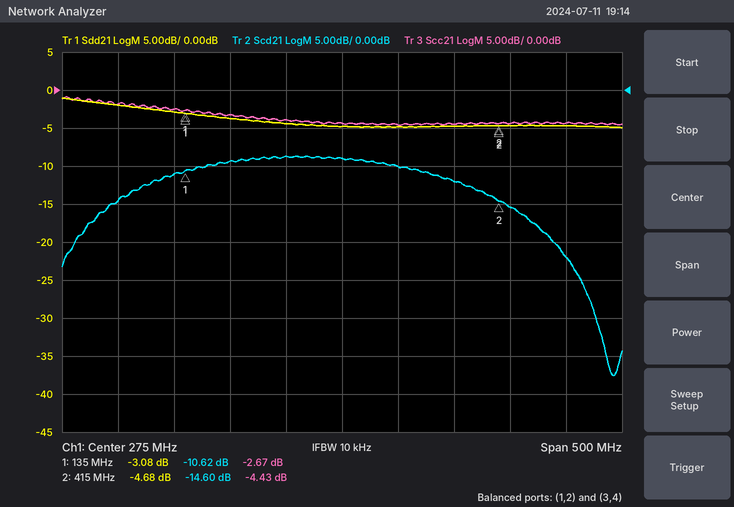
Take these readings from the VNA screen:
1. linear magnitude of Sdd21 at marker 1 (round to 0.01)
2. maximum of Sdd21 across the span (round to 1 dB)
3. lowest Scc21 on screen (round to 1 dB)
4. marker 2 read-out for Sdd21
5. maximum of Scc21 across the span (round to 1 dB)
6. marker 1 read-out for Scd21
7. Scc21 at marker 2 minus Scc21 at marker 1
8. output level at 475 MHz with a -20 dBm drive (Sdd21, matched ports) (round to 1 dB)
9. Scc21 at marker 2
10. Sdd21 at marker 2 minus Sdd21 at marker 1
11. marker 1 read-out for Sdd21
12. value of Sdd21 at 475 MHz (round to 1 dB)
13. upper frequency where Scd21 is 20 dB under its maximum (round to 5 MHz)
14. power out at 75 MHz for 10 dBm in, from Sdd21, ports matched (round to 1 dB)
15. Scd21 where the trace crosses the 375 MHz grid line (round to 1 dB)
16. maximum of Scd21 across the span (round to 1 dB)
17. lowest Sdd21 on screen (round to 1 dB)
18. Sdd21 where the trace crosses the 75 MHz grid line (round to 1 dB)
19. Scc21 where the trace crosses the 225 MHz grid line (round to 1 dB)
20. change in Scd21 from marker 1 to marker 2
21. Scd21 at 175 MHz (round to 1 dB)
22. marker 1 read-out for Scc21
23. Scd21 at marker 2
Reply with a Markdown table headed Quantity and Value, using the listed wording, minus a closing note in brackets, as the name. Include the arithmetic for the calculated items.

| Quantity | Value |
|---|---|
| linear magnitude of Sdd21 at marker 1 | 10^(-3.08/20) ≈ 0.70 |
| maximum of Sdd21 across the span | -1 dB |
| lowest Scc21 on screen | -5 dB |
| marker 2 read-out for Sdd21 | -4.68 dB |
| maximum of Scc21 across the span | -1 dB |
| marker 1 read-out for Scd21 | -10.62 dB |
| Scc21 at marker 2 minus Scc21 at marker 1 | -4.43 − (-2.67) = -1.76 dB |
| output level at 475 MHz with a -20 dBm drive (Sdd21, matched ports) | -20 dBm + (-5 dB) = -25 dBm |
| Scc21 at marker 2 | -4.43 dB |
| Sdd21 at marker 2 minus Sdd21 at marker 1 | -4.68 − (-3.08) = -1.60 dB |
| marker 1 read-out for Sdd21 | -3.08 dB |
| value of Sdd21 at 475 MHz | -5 dB |
| upper frequency where Scd21 is 20 dB under its maximum | 500 MHz |
| power out at 75 MHz for 10 dBm in, from Sdd21, ports matched | 10 dBm + (-2 dB) = 8 dBm |
| Scd21 where the trace crosses the 375 MHz grid line | -12 dB |
| maximum of Scd21 across the span | -9 dB |
| lowest Sdd21 on screen | -5 dB |
| Sdd21 where the trace crosses the 75 MHz grid line | -2 dB |
| Scc21 where the trace crosses the 225 MHz grid line | -4 dB |
| change in Scd21 from marker 1 to marker 2 | -14.6 − (-10.62) = -3.98 dB |
| Scd21 at 175 MHz | -9 dB |
| marker 1 read-out for Scc21 | -2.67 dB |
| Scd21 at marker 2 | -14.60 dB |
